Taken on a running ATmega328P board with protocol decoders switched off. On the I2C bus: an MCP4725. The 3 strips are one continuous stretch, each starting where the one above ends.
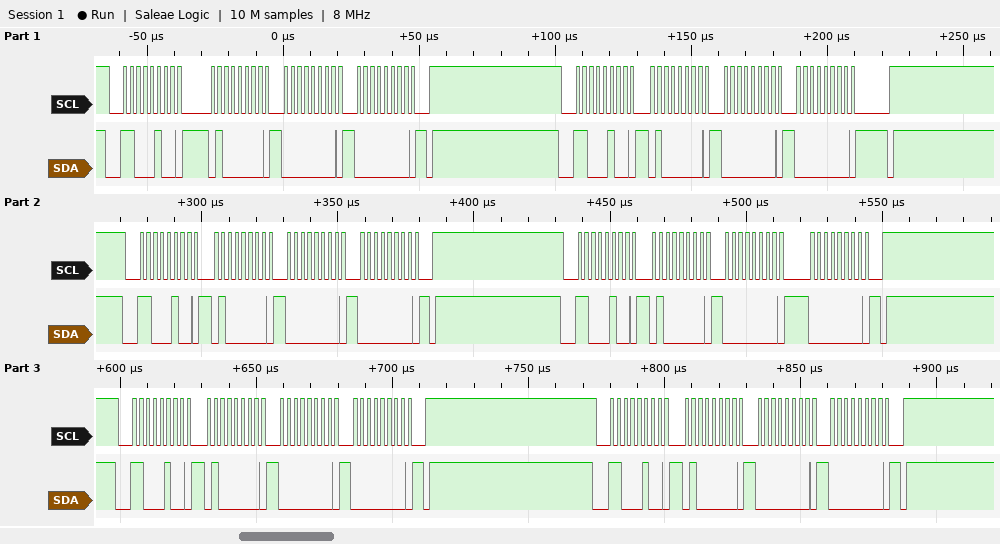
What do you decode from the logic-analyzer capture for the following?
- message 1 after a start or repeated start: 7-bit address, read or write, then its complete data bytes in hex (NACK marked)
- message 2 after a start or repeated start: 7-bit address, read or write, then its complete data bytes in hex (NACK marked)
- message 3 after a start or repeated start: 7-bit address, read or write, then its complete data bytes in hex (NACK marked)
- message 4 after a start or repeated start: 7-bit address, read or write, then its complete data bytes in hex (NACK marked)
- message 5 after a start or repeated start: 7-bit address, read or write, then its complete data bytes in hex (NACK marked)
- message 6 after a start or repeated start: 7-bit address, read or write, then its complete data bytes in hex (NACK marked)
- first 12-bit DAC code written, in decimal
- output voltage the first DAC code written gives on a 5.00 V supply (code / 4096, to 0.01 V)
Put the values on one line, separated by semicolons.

0x62 write: 40 00 00; 0x62 write: 40 00 00; 0x62 write: 40 00 00; 0x62 write: 40 00 00; 0x62 write: 40 00 00; 0x62 write: 40 00 00; 0; 0.00 V
